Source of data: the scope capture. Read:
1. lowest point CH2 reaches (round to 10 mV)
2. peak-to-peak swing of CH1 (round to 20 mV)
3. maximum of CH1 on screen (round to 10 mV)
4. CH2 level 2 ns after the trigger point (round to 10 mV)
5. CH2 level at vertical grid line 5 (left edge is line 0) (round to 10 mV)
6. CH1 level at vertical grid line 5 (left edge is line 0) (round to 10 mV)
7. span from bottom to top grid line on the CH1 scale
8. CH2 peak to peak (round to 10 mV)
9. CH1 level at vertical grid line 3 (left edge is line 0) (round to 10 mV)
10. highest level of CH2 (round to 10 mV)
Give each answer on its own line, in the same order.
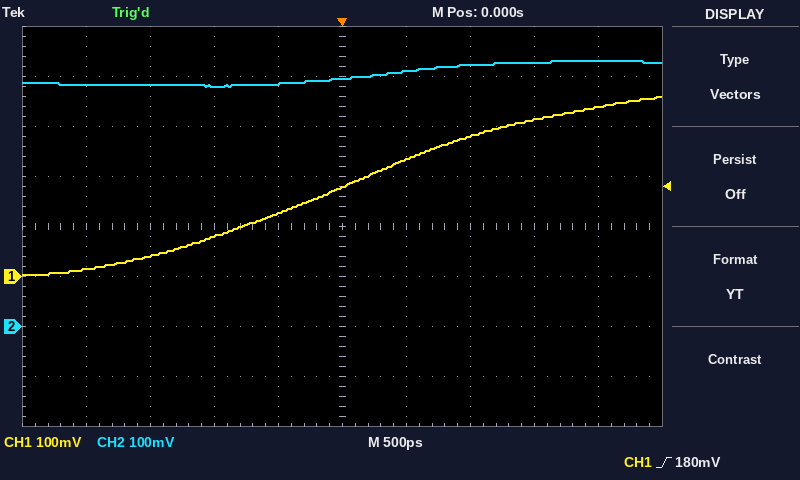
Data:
480 mV
360 mV
360 mV
530 mV
500 mV
180 mV
800 mV
50 mV
80 mV
530 mV
